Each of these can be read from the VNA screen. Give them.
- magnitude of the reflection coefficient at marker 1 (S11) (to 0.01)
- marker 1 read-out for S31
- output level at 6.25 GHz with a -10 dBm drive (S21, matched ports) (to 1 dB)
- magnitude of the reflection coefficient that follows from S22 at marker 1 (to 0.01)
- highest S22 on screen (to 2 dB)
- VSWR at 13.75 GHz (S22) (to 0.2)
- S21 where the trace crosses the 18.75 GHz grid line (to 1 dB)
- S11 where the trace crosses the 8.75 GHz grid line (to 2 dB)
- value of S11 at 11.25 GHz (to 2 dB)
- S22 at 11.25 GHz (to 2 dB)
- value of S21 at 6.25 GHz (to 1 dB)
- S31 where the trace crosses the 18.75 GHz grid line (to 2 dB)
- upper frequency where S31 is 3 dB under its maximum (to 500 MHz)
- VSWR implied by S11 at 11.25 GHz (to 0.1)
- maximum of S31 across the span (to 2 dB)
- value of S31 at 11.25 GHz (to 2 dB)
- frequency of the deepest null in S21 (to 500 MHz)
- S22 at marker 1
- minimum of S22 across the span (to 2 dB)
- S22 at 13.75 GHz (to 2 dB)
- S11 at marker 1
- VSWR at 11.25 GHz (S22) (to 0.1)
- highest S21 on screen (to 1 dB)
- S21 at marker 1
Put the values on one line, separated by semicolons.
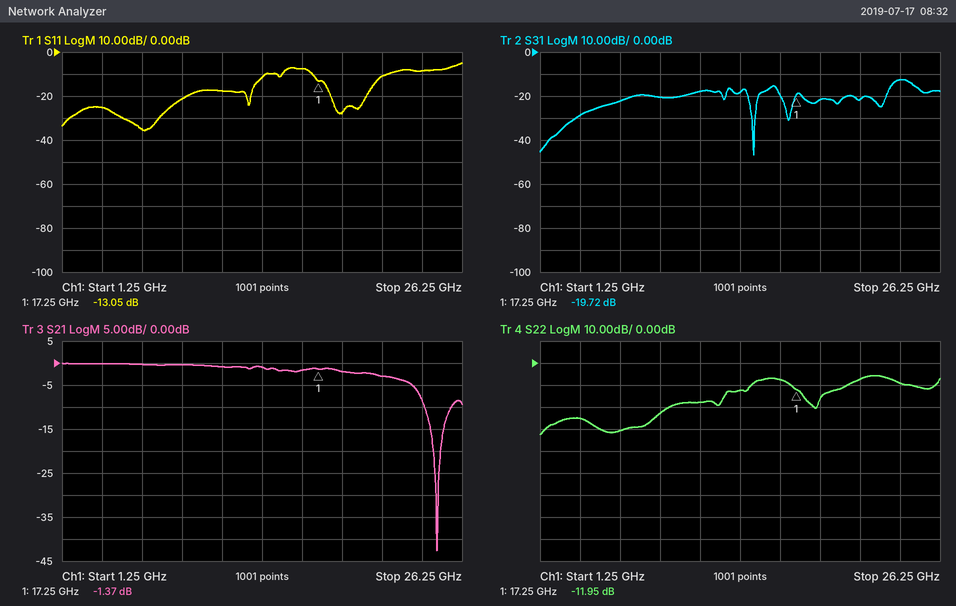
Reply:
0.22; -19.72 dB; -10 dBm; 0.25; -6 dB; 1.6; -2 dB; -22 dB; -18 dB; -18 dB; 0 dB; -22 dB; 24.5 GHz; 1.3; -12 dB; -18 dB; 24.5 GHz; -11.95 dB; -32 dB; -12 dB; -13.05 dB; 1.3; 0 dB; -1.37 dB
